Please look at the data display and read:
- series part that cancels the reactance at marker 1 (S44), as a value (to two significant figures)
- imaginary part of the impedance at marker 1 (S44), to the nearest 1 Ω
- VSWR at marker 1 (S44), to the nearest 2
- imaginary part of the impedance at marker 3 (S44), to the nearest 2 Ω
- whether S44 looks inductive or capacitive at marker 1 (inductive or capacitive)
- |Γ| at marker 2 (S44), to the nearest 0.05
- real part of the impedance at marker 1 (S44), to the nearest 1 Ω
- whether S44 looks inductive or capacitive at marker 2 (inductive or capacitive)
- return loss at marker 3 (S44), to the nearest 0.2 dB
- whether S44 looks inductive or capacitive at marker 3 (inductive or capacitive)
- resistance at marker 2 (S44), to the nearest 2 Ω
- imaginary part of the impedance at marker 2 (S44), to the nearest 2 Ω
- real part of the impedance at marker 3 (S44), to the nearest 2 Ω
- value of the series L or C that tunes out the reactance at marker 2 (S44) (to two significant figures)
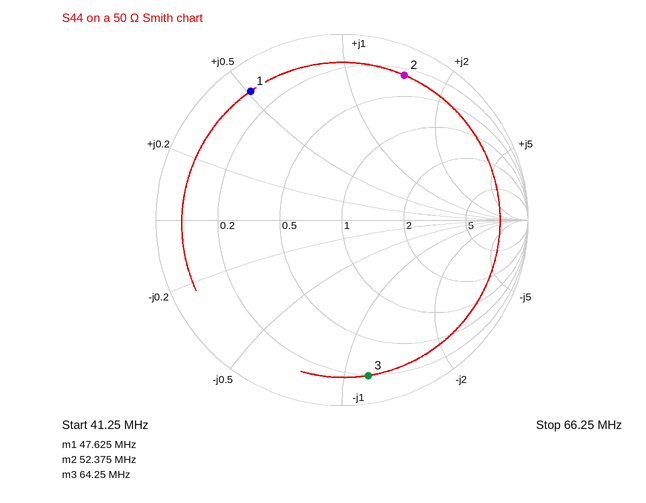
130 pF
+26 Ω
12
-58 Ω
inductive
0.85
5 Ω
inductive
1.4 dB
capacitive
14 Ω
+74 Ω
10 Ω
41 pF
